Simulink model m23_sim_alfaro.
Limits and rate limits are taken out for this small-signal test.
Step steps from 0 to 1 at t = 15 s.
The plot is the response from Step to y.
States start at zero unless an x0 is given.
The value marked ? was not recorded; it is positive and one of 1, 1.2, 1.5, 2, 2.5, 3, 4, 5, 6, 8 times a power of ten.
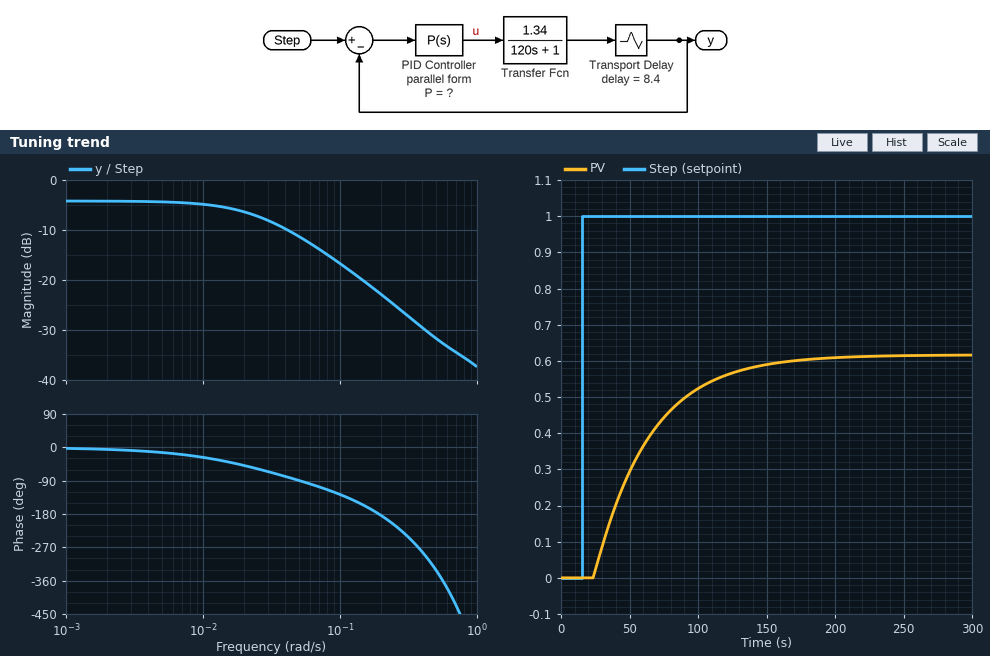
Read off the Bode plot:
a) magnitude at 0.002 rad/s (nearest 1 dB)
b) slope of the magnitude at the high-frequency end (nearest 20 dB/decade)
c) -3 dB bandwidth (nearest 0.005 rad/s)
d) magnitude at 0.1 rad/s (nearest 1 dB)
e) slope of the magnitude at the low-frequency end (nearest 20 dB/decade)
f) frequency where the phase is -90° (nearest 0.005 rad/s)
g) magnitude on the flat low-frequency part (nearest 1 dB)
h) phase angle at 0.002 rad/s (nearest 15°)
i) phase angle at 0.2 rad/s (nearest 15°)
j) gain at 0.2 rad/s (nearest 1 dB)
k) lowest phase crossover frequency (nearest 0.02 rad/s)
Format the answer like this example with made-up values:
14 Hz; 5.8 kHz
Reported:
-4 dB; -20 dB/decade; 0.025 rad/s; -17 dB; 0 dB/decade; 0.050 rad/s; -4 dB; 0°; -180°; -23 dB; 0.20 rad/s
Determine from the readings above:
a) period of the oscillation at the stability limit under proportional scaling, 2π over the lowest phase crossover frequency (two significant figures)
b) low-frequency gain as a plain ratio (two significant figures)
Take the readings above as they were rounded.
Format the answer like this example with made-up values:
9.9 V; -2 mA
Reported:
31 s; 0.63
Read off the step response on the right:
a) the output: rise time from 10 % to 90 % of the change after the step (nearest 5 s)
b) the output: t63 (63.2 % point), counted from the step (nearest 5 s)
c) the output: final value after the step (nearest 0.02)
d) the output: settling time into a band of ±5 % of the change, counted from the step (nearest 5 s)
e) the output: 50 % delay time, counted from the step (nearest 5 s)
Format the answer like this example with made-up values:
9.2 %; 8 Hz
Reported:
90 s; 50 s; 0.62; 130 s; 35 s
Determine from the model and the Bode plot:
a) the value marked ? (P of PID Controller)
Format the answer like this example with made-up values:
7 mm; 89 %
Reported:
1.2
